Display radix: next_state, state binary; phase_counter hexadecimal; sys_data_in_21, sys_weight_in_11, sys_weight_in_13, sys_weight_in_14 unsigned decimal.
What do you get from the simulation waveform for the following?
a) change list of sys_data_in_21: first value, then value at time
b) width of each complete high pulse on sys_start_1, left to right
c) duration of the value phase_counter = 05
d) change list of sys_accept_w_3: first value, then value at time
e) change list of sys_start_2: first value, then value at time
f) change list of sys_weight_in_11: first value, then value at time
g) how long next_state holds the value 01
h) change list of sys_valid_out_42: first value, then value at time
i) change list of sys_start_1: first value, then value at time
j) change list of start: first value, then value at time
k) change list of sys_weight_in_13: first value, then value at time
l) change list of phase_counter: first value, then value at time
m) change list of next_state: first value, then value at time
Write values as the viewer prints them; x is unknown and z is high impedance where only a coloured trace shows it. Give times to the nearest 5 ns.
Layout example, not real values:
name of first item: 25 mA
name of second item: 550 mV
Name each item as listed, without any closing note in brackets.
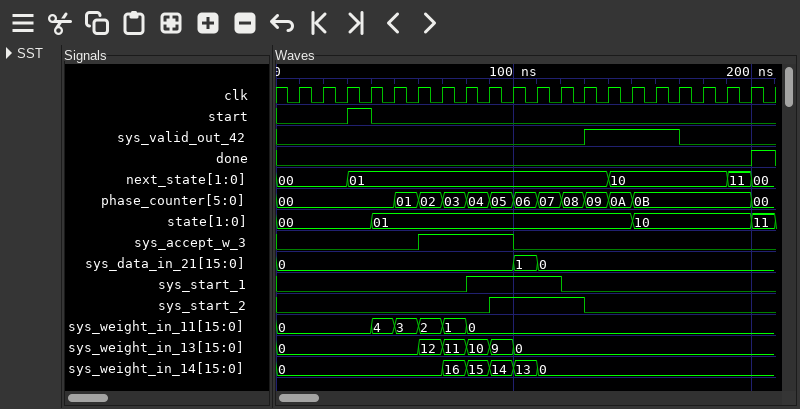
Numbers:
change list of sys_data_in_21: first value, then value at time: 0, 1 at 100 ns, 0 at 110 ns
width of each complete high pulse on sys_start_1, left to right: 40 ns
duration of the value phase_counter = 05: 10 ns
change list of sys_accept_w_3: first value, then value at time: 0, 1 at 60 ns, 0 at 100 ns
change list of sys_start_2: first value, then value at time: 0, 1 at 90 ns, 0 at 130 ns
change list of sys_weight_in_11: first value, then value at time: 0, 4 at 40 ns, 3 at 50 ns, 2 at 60 ns, 1 at 70 ns, 0 at 80 ns
how long next_state holds the value 01: 110 ns
change list of sys_valid_out_42: first value, then value at time: 0, 1 at 130 ns, 0 at 170 ns
change list of sys_start_1: first value, then value at time: 0, 1 at 80 ns, 0 at 120 ns
change list of start: first value, then value at time: 0, 1 at 30 ns, 0 at 40 ns
change list of sys_weight_in_13: first value, then value at time: 0, 12 at 60 ns, 11 at 70 ns, 10 at 80 ns, 9 at 90 ns, 0 at 100 ns
change list of phase_counter: first value, then value at time: 00, 01 at 50 ns, 02 at 60 ns, 03 at 70 ns, 04 at 80 ns, 05 at 90 ns, 06 at 100 ns, 07 at 110 ns, 08 at 120 ns, 09 at 130 ns, 0A at 140 ns, 0B at 150 ns, 00 at 200 ns
change list of next_state: first value, then value at time: 00, 01 at 30 ns, 10 at 140 ns, 11 at 190 ns, 00 at 200 ns
